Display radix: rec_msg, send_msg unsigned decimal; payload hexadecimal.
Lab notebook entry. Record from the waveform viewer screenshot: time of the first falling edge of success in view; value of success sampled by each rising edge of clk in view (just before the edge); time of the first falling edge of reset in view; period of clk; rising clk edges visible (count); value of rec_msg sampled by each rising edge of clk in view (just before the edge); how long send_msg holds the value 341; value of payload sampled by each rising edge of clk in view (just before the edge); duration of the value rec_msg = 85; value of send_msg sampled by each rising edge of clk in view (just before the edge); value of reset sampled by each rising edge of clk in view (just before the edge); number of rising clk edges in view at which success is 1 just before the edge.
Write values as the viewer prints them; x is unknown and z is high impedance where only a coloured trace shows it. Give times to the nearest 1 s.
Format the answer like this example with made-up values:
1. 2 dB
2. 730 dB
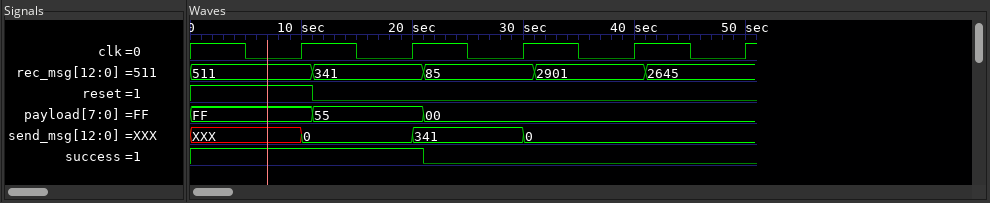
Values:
1. 21 s
2. 1 1 0 0 0
3. 11 s
4. 10 s
5. 5
6. 511, 341, 85, 2901, 2645
7. 10 s
8. FF, 55, 00, 00, 00
9. 10 s
10. XXX, 0, 341, 0, 0
11. 1 0 0 0 0
12. 2
